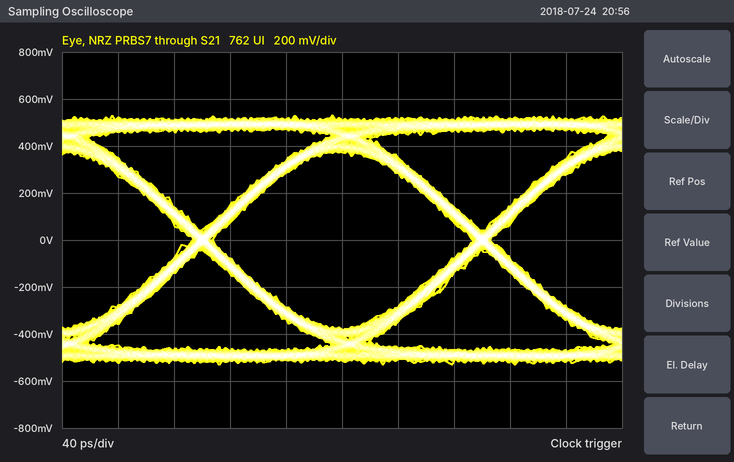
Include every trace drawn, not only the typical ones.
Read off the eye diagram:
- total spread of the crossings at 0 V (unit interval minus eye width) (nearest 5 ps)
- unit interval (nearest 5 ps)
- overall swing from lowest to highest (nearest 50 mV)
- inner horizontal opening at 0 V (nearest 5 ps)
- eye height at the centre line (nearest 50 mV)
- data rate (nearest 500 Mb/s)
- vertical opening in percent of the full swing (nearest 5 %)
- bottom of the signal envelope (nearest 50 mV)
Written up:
15 ps
200 ps
1.05 V
185 ps
750 mV
5.0 Gb/s
70 %
-550 mV
